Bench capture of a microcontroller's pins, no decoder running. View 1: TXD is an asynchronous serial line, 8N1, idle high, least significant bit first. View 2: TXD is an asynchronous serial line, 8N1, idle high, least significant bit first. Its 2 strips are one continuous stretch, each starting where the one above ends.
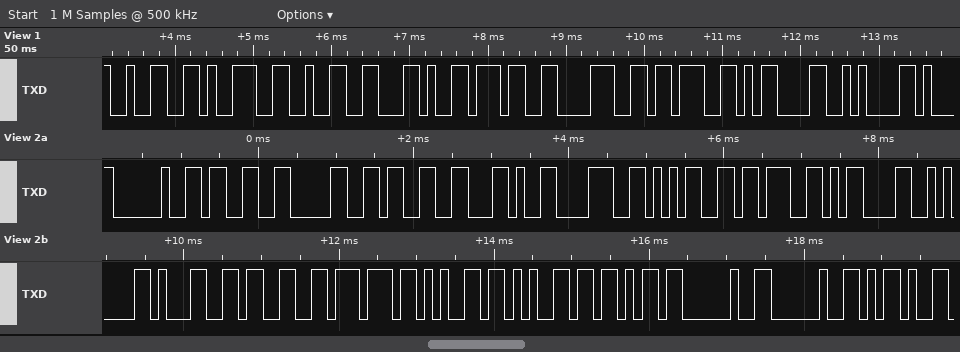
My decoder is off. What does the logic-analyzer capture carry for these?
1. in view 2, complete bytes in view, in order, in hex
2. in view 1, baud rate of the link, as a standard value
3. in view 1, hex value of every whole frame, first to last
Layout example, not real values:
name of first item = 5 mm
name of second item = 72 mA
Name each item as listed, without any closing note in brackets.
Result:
in view 2, complete bytes in view, in order, in hex = 20 33 30 33 2C 38 35 3B 0D 0A 31 33 77 65 65 6B 20 20 2D
in view 1, baud rate of the link, as a standard value = 9600 baud
in view 1, hex value of every whole frame, first to last = 32 39 32 2C 37 38 3B 0D 0A
